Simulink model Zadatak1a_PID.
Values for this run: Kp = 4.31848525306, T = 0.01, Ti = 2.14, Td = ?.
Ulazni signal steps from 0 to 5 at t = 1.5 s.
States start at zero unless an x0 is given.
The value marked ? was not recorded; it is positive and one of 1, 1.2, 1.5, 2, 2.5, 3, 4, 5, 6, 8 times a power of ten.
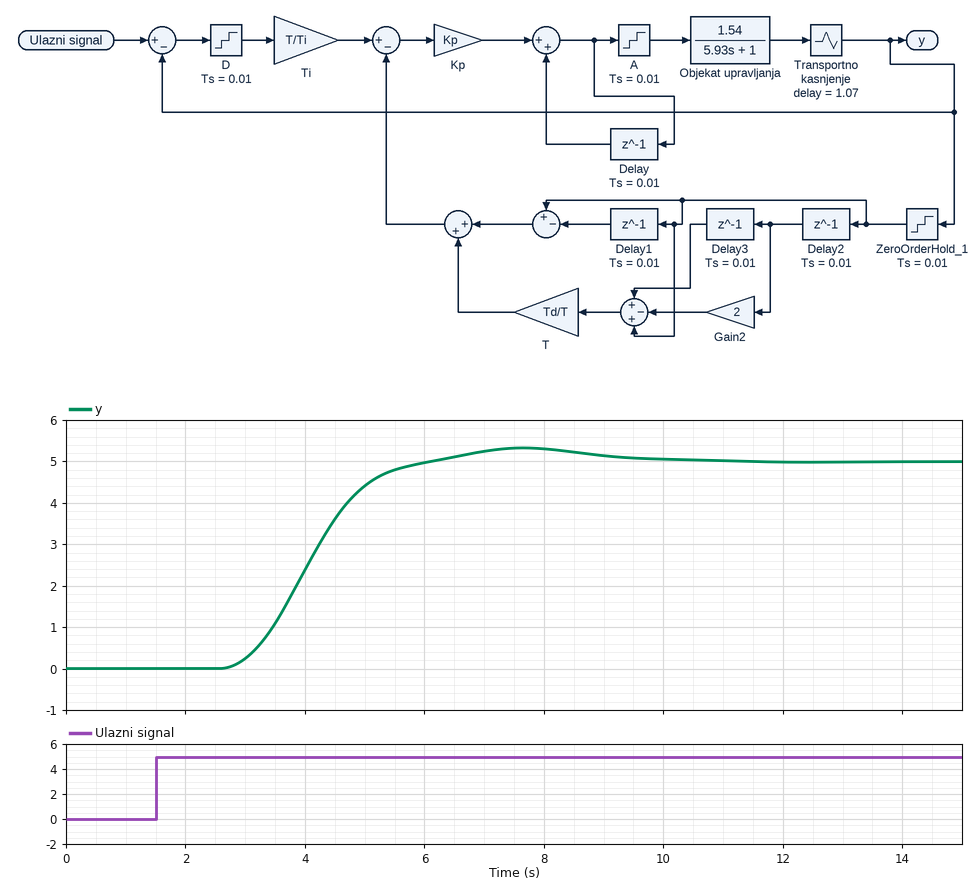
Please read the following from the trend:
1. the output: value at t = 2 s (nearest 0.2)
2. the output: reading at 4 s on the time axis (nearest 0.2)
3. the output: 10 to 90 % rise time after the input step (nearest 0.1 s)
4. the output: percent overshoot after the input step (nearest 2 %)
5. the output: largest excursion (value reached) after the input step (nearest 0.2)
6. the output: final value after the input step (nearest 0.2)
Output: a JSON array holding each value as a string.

["0.0", "2.4", "1.9 s", "6 %", "5.4", "5.0"]
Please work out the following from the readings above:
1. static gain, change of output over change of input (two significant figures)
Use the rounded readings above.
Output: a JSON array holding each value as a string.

["1.0"]
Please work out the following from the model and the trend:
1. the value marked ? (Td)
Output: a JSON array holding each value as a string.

["0.5"]
